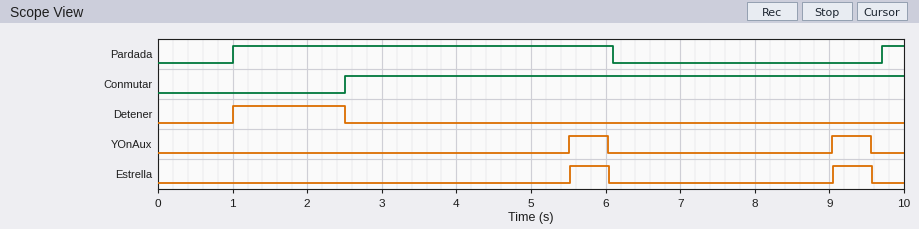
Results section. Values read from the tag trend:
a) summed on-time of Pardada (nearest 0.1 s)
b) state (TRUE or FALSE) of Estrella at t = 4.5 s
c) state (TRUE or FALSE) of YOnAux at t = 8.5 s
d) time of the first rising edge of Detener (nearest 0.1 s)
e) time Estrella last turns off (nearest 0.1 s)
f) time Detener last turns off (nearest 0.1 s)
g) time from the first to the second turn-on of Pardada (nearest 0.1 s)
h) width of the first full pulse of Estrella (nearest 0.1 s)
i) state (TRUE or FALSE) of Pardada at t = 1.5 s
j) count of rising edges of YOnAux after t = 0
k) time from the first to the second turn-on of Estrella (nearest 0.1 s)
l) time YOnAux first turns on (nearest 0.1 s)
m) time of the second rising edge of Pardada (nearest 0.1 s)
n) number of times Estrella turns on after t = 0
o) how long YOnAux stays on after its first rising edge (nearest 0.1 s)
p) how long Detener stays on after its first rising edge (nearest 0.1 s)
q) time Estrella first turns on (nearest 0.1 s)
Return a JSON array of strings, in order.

["5.4 s", "FALSE", "FALSE", "1.0 s", "9.6 s", "2.5 s", "8.7 s", "0.5 s", "TRUE", "2", "3.5 s", "5.5 s", "9.7 s", "2", "0.5 s", "1.5 s", "5.5 s"]
